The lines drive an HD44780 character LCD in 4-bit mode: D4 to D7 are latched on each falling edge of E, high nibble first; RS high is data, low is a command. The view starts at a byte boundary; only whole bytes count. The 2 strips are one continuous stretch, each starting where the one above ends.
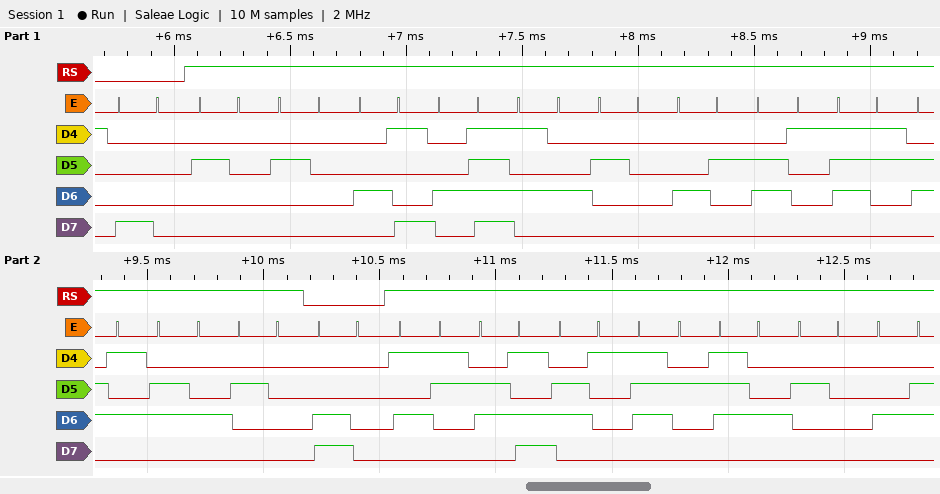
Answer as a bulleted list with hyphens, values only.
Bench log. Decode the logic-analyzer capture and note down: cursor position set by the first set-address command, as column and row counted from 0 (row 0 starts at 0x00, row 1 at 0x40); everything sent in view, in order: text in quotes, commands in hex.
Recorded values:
- column 0, row 0
- 0x80 "  IOT Based " 0xC0 "Smart F"
